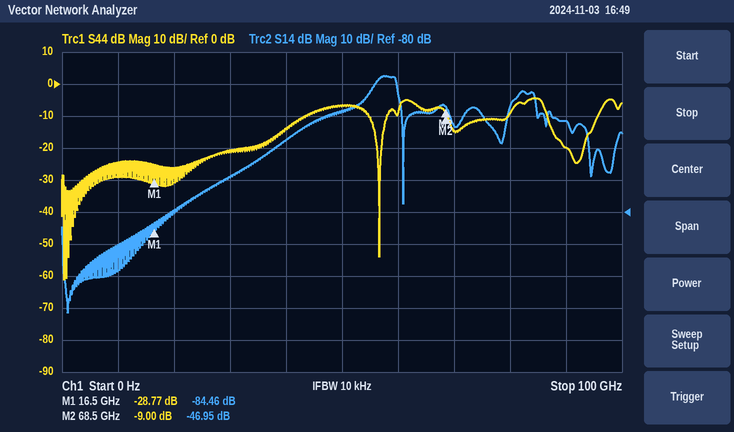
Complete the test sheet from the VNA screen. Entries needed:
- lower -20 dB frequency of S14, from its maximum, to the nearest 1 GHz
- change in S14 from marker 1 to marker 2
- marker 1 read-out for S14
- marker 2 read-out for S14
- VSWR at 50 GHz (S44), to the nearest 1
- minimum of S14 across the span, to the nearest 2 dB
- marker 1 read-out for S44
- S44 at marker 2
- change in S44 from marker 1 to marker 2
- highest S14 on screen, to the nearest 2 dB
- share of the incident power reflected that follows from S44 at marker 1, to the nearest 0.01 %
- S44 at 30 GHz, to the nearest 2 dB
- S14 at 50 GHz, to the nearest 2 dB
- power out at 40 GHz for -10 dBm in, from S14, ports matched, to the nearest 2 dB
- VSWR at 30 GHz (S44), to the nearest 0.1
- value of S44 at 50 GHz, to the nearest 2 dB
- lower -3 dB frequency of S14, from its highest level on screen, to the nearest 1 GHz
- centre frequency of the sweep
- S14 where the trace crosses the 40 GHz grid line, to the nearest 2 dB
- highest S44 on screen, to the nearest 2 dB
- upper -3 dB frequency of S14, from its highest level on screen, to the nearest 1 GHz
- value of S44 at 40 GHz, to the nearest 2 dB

40 GHz
37.51 dB
-84.46 dB
-46.95 dB
3
-112 dB
-28.77 dB
-9.00 dB
19.77 dB
-38 dB
0.13 %
-20 dB
-48 dB
-68 dBm
1.2
-6 dB
56 GHz
50 GHz
-58 dB
-4 dB
60 GHz
-14 dB
